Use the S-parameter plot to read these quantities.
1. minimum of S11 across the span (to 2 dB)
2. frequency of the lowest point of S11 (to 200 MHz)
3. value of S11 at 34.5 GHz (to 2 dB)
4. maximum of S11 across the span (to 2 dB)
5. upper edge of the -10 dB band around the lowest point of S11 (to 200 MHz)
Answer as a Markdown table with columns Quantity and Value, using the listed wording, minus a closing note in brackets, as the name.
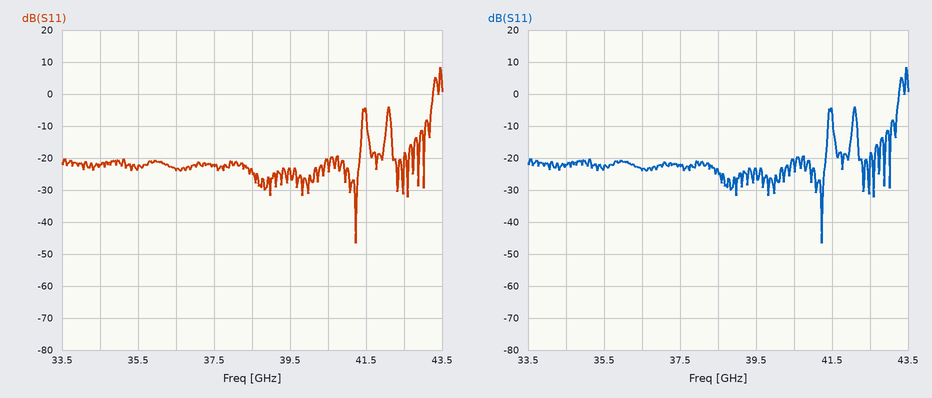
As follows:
| Quantity | Value |
|---|---|
| minimum of S11 across the span | -46 dB |
| frequency of the lowest point of S11 | 41.2 GHz |
| value of S11 at 34.5 GHz | -22 dB |
| maximum of S11 across the span | 8 dB |
| upper edge of the -10 dB band around the lowest point of S11 | 41.4 GHz |
